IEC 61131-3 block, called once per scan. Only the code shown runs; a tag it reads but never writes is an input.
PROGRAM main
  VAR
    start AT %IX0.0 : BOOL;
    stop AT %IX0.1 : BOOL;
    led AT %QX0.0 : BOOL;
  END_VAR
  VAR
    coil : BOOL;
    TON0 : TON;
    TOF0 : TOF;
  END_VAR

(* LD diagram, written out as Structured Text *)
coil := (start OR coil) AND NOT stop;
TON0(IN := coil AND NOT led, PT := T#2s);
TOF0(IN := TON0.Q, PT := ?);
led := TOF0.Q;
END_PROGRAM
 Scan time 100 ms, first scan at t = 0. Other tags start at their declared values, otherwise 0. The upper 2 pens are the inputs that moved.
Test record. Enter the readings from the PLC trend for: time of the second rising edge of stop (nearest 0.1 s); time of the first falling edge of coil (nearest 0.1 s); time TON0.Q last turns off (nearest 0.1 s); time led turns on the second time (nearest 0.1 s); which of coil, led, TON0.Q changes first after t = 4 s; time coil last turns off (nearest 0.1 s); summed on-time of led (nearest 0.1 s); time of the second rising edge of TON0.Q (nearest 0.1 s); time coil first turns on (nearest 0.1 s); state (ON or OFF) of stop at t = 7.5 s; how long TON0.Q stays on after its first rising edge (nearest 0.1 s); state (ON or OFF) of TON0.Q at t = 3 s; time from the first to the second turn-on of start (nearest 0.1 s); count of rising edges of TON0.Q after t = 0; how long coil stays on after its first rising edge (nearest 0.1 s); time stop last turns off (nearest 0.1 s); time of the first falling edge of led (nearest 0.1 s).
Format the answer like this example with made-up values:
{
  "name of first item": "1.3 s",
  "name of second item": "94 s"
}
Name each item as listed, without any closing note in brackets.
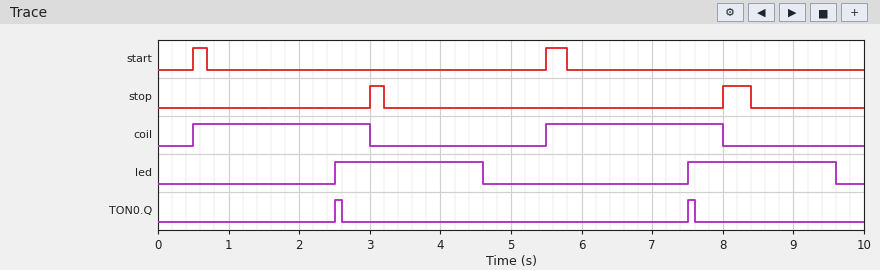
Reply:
{
  "time of the second rising edge of stop": "8.0 s",
  "time of the first falling edge of coil": "3.0 s",
  "time TON0.Q last turns off": "7.6 s",
  "time led turns on the second time": "7.5 s",
  "which of coil, led, TON0.Q changes first after t = 4 s": "led",
  "time coil last turns off": "8.0 s",
  "summed on-time of led": "4.2 s",
  "time of the second rising edge of TON0.Q": "7.5 s",
  "time coil first turns on": "0.5 s",
  "state (ON or OFF) of stop at t = 7.5 s": "OFF",
  "how long TON0.Q stays on after its first rising edge": "0.1 s",
  "state (ON or OFF) of TON0.Q at t = 3 s": "OFF",
  "time from the first to the second turn-on of start": "5.0 s",
  "count of rising edges of TON0.Q after t = 0": "2",
  "how long coil stays on after its first rising edge": "2.5 s",
  "time stop last turns off": "8.4 s",
  "time of the first falling edge of led": "4.6 s"
}
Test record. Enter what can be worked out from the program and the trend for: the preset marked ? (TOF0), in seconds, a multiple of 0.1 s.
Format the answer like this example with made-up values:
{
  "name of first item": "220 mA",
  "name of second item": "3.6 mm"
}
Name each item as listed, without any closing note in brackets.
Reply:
{
  "the preset marked ? (TOF0), in seconds, a multiple of 0.1 s": "2.0 s"
}
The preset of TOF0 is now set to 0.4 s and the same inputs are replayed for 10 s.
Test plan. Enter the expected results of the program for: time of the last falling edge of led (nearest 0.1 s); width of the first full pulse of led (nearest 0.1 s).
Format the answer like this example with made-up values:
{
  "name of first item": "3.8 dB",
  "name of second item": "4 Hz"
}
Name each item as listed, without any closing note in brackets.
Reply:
{
  "time of the last falling edge of led": "8.0 s",
  "width of the first full pulse of led": "0.5 s"
}
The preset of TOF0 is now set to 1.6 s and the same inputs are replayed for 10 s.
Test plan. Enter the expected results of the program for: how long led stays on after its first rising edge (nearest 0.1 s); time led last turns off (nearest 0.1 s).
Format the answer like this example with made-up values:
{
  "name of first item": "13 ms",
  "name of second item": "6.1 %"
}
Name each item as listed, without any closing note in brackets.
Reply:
{
  "how long led stays on after its first rising edge": "1.7 s",
  "time led last turns off": "9.2 s"
}
